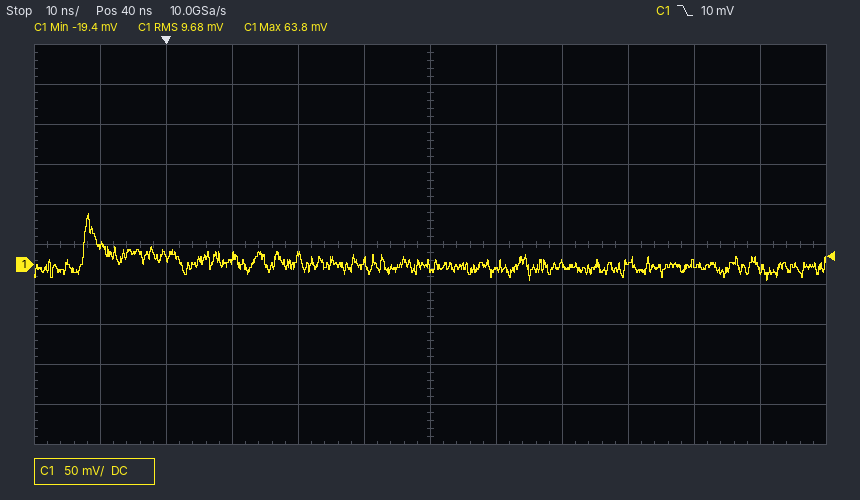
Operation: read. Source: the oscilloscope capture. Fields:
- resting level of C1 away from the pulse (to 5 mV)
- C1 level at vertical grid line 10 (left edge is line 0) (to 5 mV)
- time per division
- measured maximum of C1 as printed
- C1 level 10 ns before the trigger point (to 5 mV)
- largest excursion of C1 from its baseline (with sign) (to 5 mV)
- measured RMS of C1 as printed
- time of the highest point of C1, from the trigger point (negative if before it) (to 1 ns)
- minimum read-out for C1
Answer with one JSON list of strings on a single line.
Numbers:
["0 mV", "0 mV", "10 ns", "63.8 mV", "25 mV", "+65 mV", "9.68 mV", "-12 ns", "-19.4 mV"]
